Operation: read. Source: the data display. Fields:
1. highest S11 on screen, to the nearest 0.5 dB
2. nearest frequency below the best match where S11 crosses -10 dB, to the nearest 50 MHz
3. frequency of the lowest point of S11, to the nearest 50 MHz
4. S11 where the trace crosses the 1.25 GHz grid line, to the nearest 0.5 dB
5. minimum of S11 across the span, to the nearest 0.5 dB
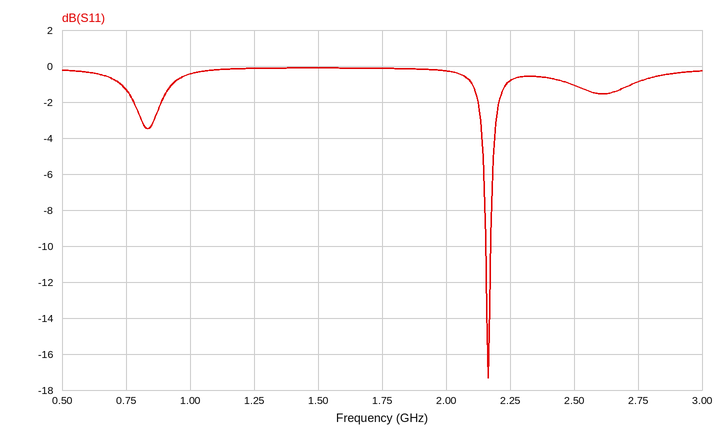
0.0 dB
2.15 GHz
2.15 GHz
0.0 dB
-17.5 dB
